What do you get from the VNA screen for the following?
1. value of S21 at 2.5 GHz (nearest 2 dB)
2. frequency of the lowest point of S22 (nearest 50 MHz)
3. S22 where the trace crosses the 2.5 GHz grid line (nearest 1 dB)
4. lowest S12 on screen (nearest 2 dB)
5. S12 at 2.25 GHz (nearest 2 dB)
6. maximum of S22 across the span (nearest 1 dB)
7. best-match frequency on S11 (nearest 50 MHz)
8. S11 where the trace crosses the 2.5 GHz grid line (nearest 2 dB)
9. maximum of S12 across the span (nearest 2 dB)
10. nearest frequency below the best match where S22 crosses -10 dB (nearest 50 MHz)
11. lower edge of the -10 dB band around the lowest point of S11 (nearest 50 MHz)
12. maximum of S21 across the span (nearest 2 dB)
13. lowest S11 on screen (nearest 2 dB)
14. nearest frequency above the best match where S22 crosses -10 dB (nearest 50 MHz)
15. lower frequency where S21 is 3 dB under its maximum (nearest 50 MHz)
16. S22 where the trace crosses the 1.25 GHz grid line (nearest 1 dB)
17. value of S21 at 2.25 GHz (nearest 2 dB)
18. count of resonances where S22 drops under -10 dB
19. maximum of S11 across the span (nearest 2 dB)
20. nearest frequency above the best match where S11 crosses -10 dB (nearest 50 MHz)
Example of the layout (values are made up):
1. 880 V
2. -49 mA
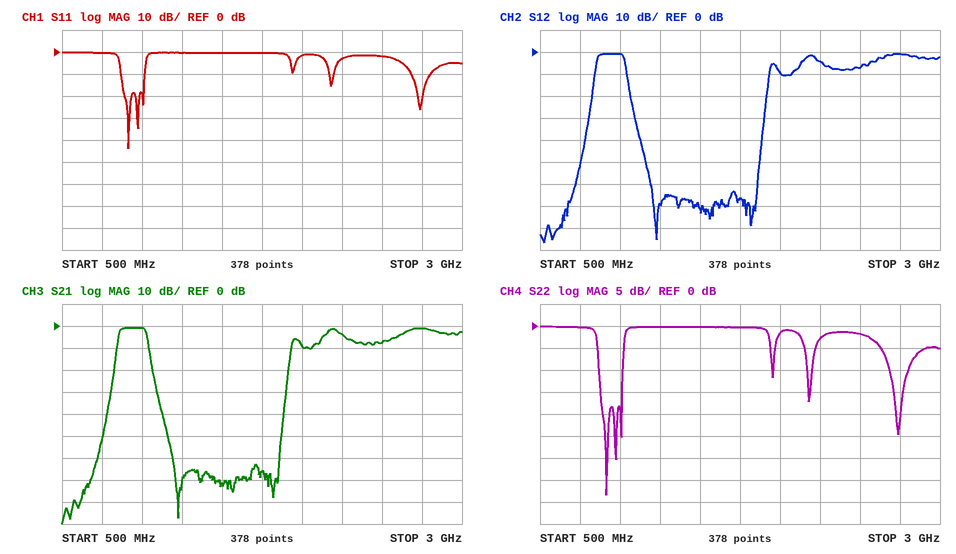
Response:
1. -8 dB
2. 900 MHz
3. -2 dB
4. -86 dB
5. -4 dB
6. 0 dB
7. 900 MHz
8. -2 dB
9. 0 dB
10. 850 MHz
11. 850 MHz
12. 0 dB
13. -44 dB
14. 1.00 GHz
15. 850 MHz
16. 0 dB
17. -4 dB
18. 6
19. 0 dB
20. 1.00 GHz
